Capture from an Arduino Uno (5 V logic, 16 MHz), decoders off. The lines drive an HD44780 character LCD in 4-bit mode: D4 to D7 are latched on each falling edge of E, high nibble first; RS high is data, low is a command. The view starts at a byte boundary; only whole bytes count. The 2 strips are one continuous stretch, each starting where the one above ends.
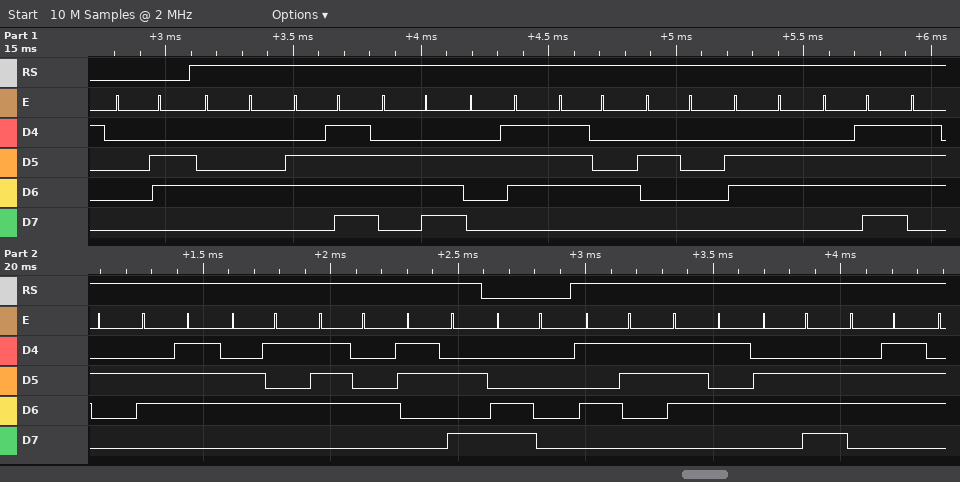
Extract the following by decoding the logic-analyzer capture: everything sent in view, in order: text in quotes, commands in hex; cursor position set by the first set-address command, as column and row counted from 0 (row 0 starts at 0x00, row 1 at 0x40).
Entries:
0x06 "Don't forget:" 0xC0 "Sung"
column 0, row 1
